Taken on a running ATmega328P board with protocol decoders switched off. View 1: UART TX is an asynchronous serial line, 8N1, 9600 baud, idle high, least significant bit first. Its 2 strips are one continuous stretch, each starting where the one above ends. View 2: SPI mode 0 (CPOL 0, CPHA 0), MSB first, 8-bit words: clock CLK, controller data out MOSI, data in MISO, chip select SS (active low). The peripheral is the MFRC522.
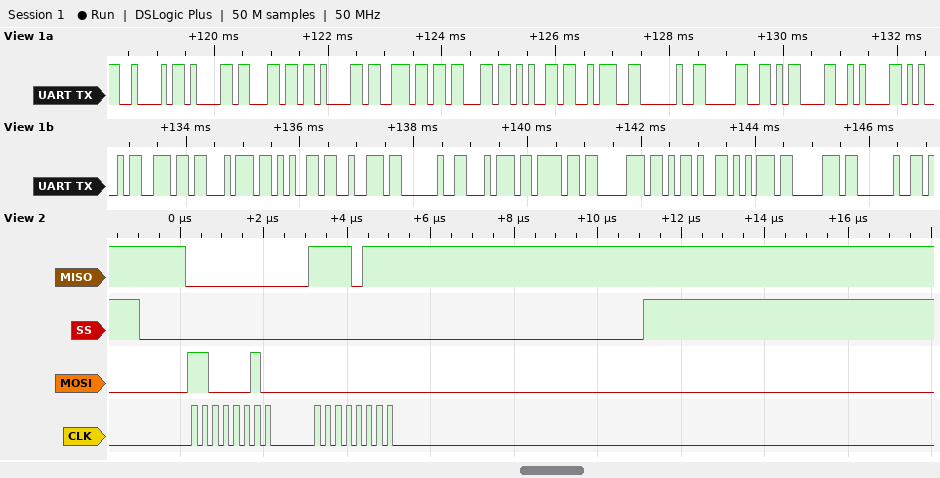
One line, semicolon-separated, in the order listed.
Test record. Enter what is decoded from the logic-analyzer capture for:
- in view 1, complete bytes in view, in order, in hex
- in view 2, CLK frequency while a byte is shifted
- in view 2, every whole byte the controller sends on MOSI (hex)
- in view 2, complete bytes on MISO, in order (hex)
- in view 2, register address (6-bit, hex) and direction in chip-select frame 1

0x42 0x61 0x6C 0x61 0x6E 0x63 0x65 0x3A 0x20 0x30 0x0D 0x0A 0x45 0x6E 0x74 0x65 0x72 0x20 0x74 0x6F 0x70 0x2D 0x75 0x70 0x20; 4 MHz; 0xC2 0x00; 0x00 0xF7; 0x21 read
